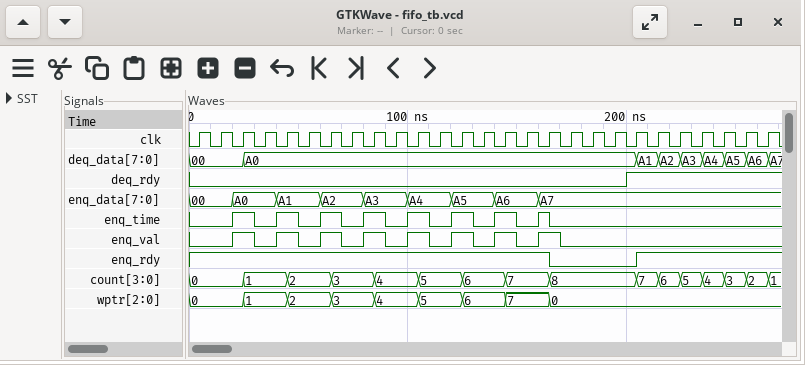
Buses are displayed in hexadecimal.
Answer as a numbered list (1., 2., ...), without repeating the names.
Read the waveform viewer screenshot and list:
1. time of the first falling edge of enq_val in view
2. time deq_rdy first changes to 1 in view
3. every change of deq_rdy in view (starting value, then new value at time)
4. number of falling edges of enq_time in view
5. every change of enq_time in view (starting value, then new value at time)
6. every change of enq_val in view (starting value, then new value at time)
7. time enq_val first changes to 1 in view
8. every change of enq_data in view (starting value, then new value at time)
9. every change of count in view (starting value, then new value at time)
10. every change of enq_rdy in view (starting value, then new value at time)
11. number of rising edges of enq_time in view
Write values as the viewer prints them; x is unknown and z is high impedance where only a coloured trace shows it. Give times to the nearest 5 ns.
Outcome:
1. 30 ns
2. 200 ns
3. 0, 1 at 200 ns
4. 8
5. 0, 1 at 20 ns, 0 at 30 ns, 1 at 40 ns, 0 at 50 ns, 1 at 60 ns, 0 at 70 ns, 1 at 80 ns, 0 at 90 ns, 1 at 100 ns, 0 at 110 ns, 1 at 120 ns, 0 at 130 ns, 1 at 140 ns, 0 at 150 ns, 1 at 160 ns, 0 at 165 ns
6. 0, 1 at 20 ns, 0 at 30 ns, 1 at 40 ns, 0 at 50 ns, 1 at 60 ns, 0 at 70 ns, 1 at 80 ns, 0 at 90 ns, 1 at 100 ns, 0 at 110 ns, 1 at 120 ns, 0 at 130 ns, 1 at 140 ns, 0 at 150 ns, 1 at 160 ns, 0 at 170 ns
7. 20 ns
8. 00, A0 at 20 ns, A1 at 40 ns, A2 at 60 ns, A3 at 80 ns, A4 at 100 ns, A5 at 120 ns, A6 at 140 ns, A7 at 160 ns
9. 0, 1 at 25 ns, 2 at 45 ns, 3 at 65 ns, 4 at 85 ns, 5 at 105 ns, 6 at 125 ns, 7 at 145 ns, 8 at 165 ns, 7 at 205 ns, 6 at 215 ns, 5 at 225 ns, 4 at 235 ns, 3 at 245 ns, 2 at 255 ns, 1 at 265 ns
10. 1, 0 at 165 ns, 1 at 205 ns
11. 8
